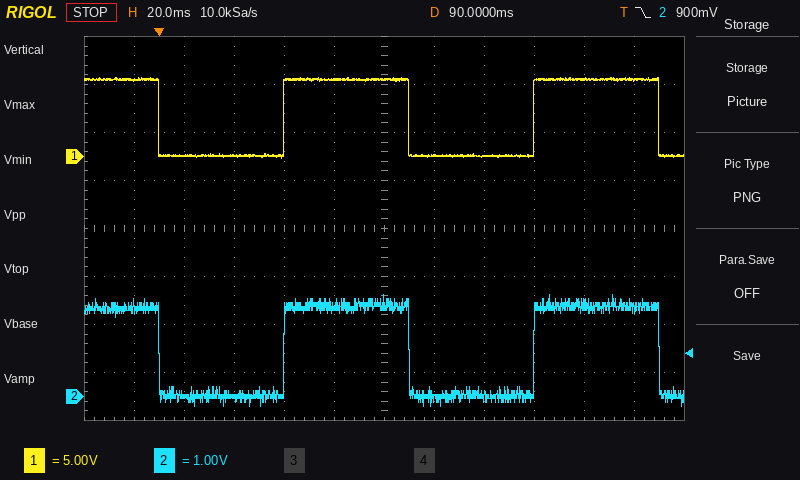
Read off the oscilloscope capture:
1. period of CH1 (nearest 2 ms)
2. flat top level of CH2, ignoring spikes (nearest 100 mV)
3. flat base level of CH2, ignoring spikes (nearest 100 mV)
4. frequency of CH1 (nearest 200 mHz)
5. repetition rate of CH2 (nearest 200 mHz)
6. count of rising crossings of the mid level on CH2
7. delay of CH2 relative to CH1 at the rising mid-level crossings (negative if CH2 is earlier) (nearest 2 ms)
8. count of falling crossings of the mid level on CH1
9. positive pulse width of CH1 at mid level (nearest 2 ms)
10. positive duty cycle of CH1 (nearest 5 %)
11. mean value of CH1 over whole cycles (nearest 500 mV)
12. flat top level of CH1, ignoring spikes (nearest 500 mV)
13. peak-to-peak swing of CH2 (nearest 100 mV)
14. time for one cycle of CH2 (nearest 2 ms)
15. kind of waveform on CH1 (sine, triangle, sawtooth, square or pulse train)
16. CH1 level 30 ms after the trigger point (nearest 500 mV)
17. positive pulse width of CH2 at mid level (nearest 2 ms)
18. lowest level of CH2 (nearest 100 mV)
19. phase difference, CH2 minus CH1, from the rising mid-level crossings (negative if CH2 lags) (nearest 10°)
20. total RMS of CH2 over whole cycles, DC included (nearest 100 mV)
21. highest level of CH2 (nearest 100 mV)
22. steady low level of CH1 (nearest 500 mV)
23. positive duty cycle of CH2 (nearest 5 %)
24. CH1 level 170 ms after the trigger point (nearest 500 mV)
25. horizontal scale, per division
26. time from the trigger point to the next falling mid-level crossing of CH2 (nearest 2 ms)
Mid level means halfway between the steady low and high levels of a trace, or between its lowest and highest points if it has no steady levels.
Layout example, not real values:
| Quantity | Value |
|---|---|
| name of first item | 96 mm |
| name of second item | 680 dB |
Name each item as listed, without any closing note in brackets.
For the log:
| Quantity | Value |
|---|---|
| period of CH1 | 100 ms |
| flat top level of CH2, ignoring spikes | 1.9 V |
| flat base level of CH2, ignoring spikes | 0.0 V |
| frequency of CH1 | 10.0 Hz |
| repetition rate of CH2 | 10.0 Hz |
| count of rising crossings of the mid level on CH2 | 2 |
| delay of CH2 relative to CH1 at the rising mid-level crossings (negative if CH2 is earlier) | 0 ms |
| count of falling crossings of the mid level on CH1 | 3 |
| positive pulse width of CH1 at mid level | 50 ms |
| positive duty cycle of CH1 | 50 % |
| mean value of CH1 over whole cycles | 4.0 V |
| flat top level of CH1, ignoring spikes | 8.0 V |
| peak-to-peak swing of CH2 | 2.3 V |
| time for one cycle of CH2 | 100 ms |
| kind of waveform on CH1 | square |
| CH1 level 30 ms after the trigger point | 0.0 V |
| positive pulse width of CH2 at mid level | 50 ms |
| lowest level of CH2 | -200 mV |
| phase difference, CH2 minus CH1, from the rising mid-level crossings (negative if CH2 lags) | 0° |
| total RMS of CH2 over whole cycles, DC included | 1.3 V |
| highest level of CH2 | 2.1 V |
| steady low level of CH1 | 0.0 V |
| positive duty cycle of CH2 | 50 % |
| CH1 level 170 ms after the trigger point | 8.0 V |
| horizontal scale, per division | 20 ms |
| time from the trigger point to the next falling mid-level crossing of CH2 | 100 ms |
